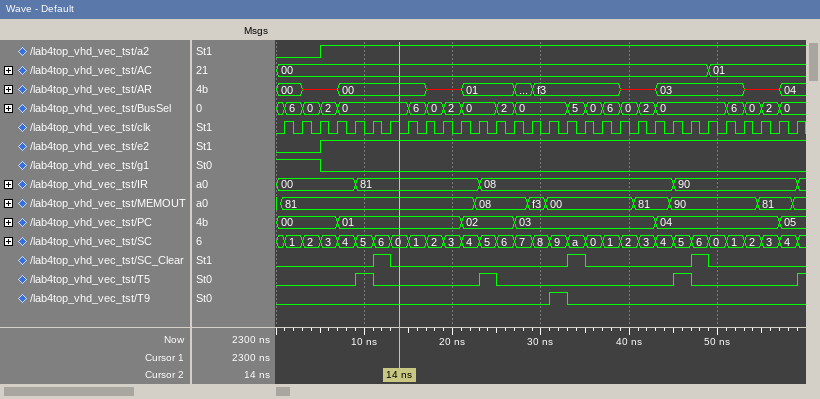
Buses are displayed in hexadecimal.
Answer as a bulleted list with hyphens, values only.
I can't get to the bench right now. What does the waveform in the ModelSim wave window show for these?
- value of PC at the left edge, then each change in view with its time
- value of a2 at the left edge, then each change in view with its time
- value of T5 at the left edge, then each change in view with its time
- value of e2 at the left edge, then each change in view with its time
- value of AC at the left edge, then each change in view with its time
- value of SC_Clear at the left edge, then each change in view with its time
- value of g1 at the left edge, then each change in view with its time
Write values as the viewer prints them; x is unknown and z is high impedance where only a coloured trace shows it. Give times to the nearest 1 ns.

- 00, 01 at 7 ns, 02 at 21 ns, 03 at 27 ns, 04 at 43 ns, 05 at 57 ns
- 0, 1 at 5 ns
- 0, 1 at 9 ns, 0 at 11 ns, 1 at 23 ns, 0 at 25 ns, 1 at 45 ns, 0 at 47 ns, 1 at 59 ns
- 0, 1 at 5 ns
- 00, 01 at 49 ns
- 0, 1 at 11 ns, 0 at 13 ns, 1 at 33 ns, 0 at 35 ns, 1 at 47 ns, 0 at 49 ns
- 1, 0 at 5 ns
